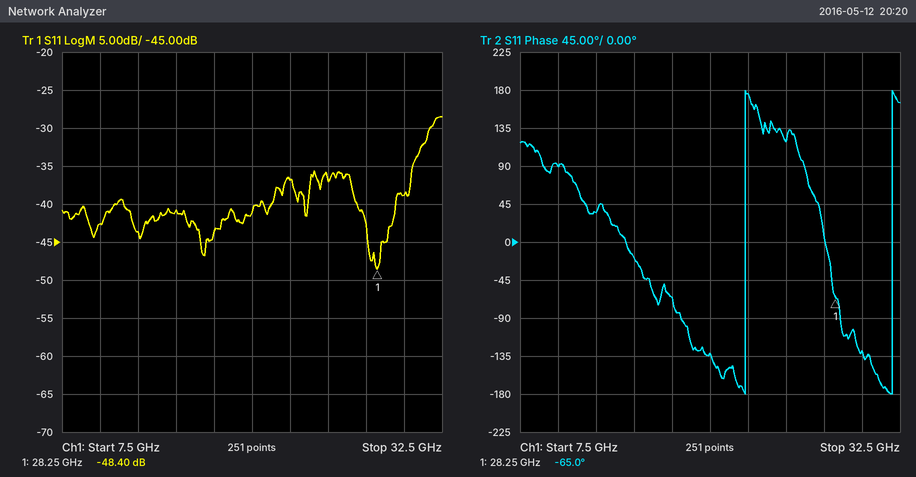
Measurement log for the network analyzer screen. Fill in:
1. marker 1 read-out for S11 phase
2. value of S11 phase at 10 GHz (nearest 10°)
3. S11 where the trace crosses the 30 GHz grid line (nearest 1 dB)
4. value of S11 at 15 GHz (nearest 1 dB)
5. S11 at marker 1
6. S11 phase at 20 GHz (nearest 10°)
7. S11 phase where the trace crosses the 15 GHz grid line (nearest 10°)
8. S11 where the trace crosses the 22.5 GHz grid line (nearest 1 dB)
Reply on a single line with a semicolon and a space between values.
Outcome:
-65.0°; 90°; -39 dB; -41 dB; -48.40 dB; -130°; -20°; -37 dB
